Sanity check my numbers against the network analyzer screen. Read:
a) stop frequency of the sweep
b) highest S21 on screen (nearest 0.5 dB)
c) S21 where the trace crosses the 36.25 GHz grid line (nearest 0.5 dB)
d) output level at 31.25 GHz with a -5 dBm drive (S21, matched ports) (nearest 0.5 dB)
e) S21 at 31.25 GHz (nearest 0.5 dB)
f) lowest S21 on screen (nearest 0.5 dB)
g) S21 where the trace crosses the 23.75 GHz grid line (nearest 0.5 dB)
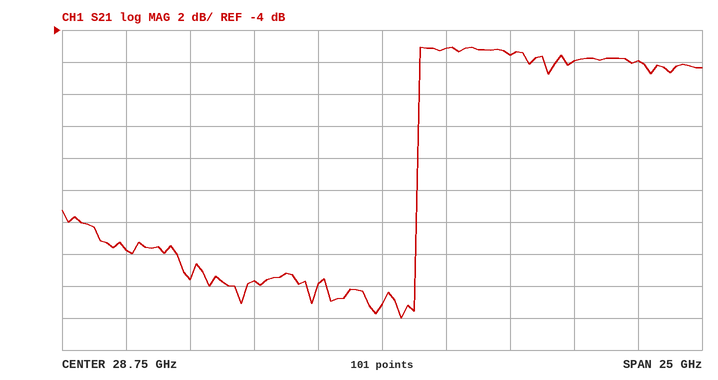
41.25 GHz
-5.0 dB
-6.0 dB
-10.0 dBm
-5.0 dB
-22.0 dB
-19.5 dB
